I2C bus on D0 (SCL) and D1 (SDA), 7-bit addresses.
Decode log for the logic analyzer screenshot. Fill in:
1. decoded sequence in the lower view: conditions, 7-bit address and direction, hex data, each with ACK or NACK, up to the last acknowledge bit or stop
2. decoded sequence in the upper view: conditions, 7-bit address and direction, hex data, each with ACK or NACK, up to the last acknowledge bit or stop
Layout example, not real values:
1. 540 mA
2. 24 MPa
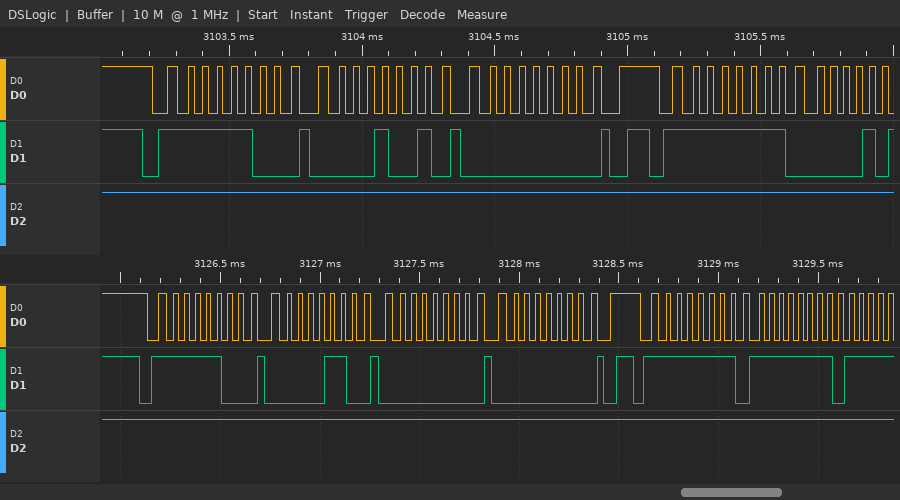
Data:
1. start, address 7E write ACK, 06 ACK, 00 ACK, 00 ACK, stop, start, address 7F read ACK, FF ACK
2. start, address 7E write ACK, 09 ACK, 00 ACK, stop, start, address 7F read ACK
